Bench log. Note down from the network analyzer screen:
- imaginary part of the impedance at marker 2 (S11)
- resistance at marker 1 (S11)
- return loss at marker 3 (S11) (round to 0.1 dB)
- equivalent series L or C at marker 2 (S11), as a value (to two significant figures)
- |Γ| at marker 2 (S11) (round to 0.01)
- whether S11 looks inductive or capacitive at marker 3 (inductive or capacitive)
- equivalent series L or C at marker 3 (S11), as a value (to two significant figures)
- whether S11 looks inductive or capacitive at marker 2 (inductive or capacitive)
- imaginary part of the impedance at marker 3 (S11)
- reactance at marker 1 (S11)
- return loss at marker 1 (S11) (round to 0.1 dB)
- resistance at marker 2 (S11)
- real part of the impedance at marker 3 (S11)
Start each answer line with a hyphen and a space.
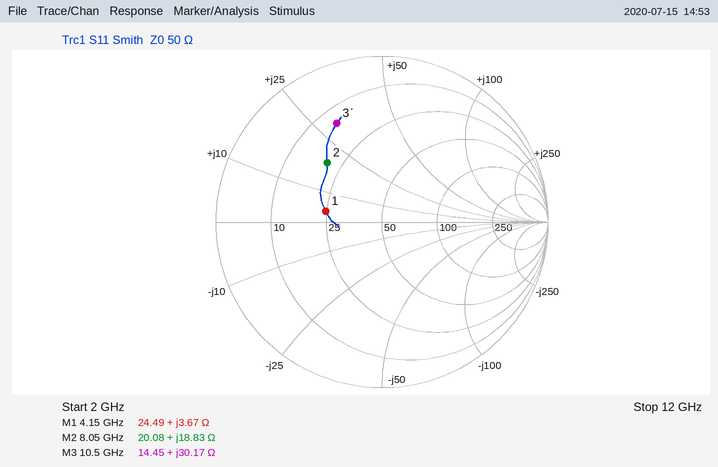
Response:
- +18.83 Ω
- 24.49 Ω
- 3.7 dB
- 370 pH
- 0.49
- inductive
- 460 pH
- inductive
- +30.17 Ω
- +3.67 Ω
- 9.2 dB
- 20.08 Ω
- 14.45 Ω
